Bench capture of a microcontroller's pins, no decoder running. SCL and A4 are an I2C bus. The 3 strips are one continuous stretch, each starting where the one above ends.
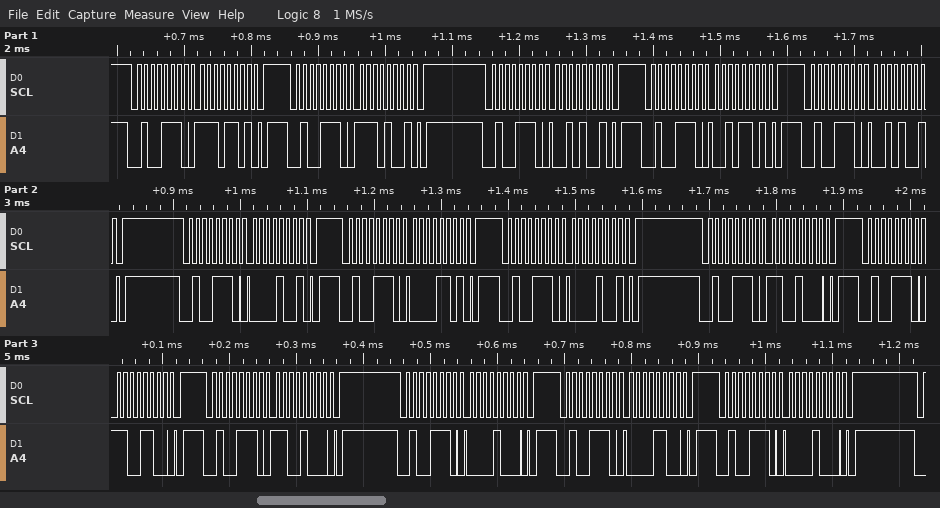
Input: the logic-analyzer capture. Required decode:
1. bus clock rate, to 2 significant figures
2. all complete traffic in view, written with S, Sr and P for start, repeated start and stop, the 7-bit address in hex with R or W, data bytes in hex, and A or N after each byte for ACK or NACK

100 kHz
S 27W A ED A P S 27W A E9 A P S 27W A 29 A P S 27W A 2D A P S 27W A 29 A P S 27W A 09 A P S 27W A 0D A P S 27W A 09 A P S 27W A C8 A P S 27W A CC A P S 27W A C8 A P S 27W A 08 A P S 27W A 0C A P S 27W A 08 A P
